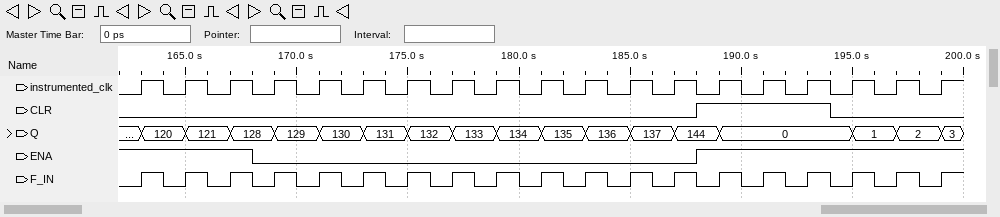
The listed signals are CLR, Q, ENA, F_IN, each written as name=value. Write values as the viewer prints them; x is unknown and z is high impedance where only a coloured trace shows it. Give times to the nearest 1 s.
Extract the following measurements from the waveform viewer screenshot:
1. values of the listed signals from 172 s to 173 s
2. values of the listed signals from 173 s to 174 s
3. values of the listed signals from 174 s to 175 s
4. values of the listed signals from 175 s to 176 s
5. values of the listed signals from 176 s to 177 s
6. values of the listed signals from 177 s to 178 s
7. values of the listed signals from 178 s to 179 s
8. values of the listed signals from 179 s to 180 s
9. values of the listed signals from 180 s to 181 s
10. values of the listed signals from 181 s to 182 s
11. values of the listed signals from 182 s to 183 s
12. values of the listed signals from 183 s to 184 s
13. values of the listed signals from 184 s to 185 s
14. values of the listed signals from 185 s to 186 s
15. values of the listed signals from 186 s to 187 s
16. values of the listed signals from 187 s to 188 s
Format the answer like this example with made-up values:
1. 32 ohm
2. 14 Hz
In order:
1. CLR=0, Q=130, ENA=0, F_IN=0
2. CLR=0, Q=131, ENA=0, F_IN=1
3. CLR=0, Q=131, ENA=0, F_IN=0
4. CLR=0, Q=132, ENA=0, F_IN=1
5. CLR=0, Q=132, ENA=0, F_IN=0
6. CLR=0, Q=133, ENA=0, F_IN=1
7. CLR=0, Q=133, ENA=0, F_IN=0
8. CLR=0, Q=134, ENA=0, F_IN=1
9. CLR=0, Q=134, ENA=0, F_IN=0
10. CLR=0, Q=135, ENA=0, F_IN=1
11. CLR=0, Q=135, ENA=0, F_IN=0
12. CLR=0, Q=136, ENA=0, F_IN=1
13. CLR=0, Q=136, ENA=0, F_IN=0
14. CLR=0, Q=137, ENA=0, F_IN=1
15. CLR=0, Q=137, ENA=0, F_IN=0
16. CLR=0, Q=144, ENA=0, F_IN=1
